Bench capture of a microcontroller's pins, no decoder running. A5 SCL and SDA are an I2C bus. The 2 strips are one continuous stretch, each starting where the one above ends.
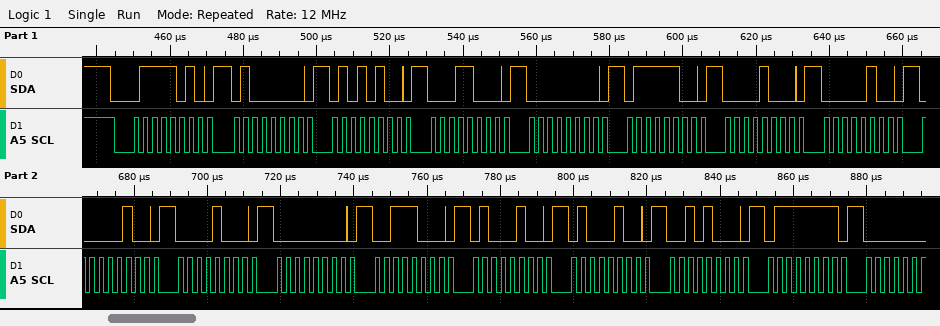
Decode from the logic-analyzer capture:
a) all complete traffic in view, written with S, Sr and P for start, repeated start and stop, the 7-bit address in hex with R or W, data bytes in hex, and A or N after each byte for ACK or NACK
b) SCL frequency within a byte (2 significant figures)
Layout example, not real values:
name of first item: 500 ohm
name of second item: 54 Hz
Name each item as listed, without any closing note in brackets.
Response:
all complete traffic in view, written with S, Sr and P for start, repeated start and stop, the 7-bit address in hex with R or W, data bytes in hex, and A or N after each byte for ACK or NACK: S 3DW A 40 A 54 A 18 A 00 A 7C A 08 A 04 A 04 A 08 A 00 A 38 A 44 A 44 A 28 A 7F A
SCL frequency within a byte: 400 kHz
